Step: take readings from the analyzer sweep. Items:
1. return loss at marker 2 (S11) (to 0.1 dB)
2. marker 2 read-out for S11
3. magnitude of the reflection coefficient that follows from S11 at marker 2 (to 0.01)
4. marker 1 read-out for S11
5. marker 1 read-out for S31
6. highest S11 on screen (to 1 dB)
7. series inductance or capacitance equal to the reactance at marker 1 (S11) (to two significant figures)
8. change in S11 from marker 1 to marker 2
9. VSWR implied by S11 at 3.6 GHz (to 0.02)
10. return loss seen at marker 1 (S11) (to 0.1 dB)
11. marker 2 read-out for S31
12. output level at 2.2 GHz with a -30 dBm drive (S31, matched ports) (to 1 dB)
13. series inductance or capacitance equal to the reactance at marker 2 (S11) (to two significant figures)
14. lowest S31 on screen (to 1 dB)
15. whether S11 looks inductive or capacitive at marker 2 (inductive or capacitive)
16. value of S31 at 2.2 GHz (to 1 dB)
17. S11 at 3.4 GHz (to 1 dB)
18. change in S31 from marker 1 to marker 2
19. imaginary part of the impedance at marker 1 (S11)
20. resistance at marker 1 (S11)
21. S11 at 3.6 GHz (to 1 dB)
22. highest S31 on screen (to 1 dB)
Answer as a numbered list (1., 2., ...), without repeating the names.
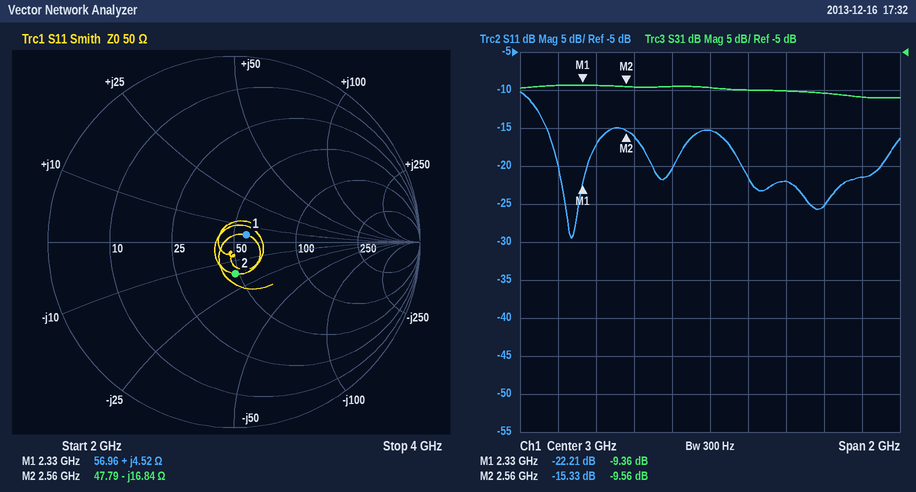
1. 15.3 dB
2. -15.33 dB
3. 0.17
4. -22.21 dB
5. -9.36 dB
6. -10 dB
7. 310 pH
8. 6.88 dB
9. 1.12
10. 22.2 dB
11. -9.56 dB
12. -39 dBm
13. 3.7 pF
14. -11 dB
15. capacitive
16. -9 dB
17. -22 dB
18. -0.20 dB
19. +4.52 Ω
20. 56.96 Ω
21. -25 dB
22. -9 dB
